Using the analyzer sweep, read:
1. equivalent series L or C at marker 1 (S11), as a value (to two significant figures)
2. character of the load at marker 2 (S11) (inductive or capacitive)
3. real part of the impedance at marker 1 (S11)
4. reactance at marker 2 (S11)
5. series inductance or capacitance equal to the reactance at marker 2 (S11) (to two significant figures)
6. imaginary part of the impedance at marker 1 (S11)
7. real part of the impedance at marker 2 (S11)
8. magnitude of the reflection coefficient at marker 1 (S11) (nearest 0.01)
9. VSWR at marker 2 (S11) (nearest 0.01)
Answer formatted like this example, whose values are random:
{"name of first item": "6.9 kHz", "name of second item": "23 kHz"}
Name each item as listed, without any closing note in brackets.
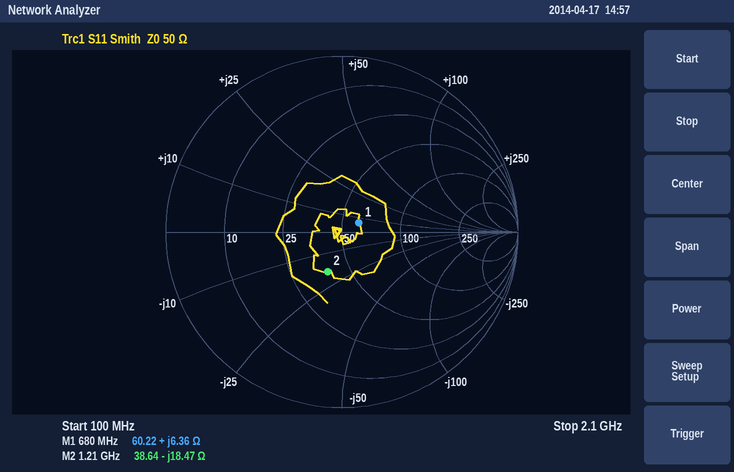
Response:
{"equivalent series L or C at marker 1 (S11), as a value": "1.5 nH", "character of the load at marker 2 (S11)": "capacitive", "real part of the impedance at marker 1": "60.22 Ω", "reactance at marker 2": "-18.47 Ω", "series inductance or capacitance equal to the reactance at marker 2 (S11)": "7.1 pF", "imaginary part of the impedance at marker 1": "+6.36 Ω", "real part of the impedance at marker 2": "38.64 Ω", "magnitude of the reflection coefficient at marker 1 (S11)": "0.11", "VSWR at marker 2 (S11)": "1.63"}
